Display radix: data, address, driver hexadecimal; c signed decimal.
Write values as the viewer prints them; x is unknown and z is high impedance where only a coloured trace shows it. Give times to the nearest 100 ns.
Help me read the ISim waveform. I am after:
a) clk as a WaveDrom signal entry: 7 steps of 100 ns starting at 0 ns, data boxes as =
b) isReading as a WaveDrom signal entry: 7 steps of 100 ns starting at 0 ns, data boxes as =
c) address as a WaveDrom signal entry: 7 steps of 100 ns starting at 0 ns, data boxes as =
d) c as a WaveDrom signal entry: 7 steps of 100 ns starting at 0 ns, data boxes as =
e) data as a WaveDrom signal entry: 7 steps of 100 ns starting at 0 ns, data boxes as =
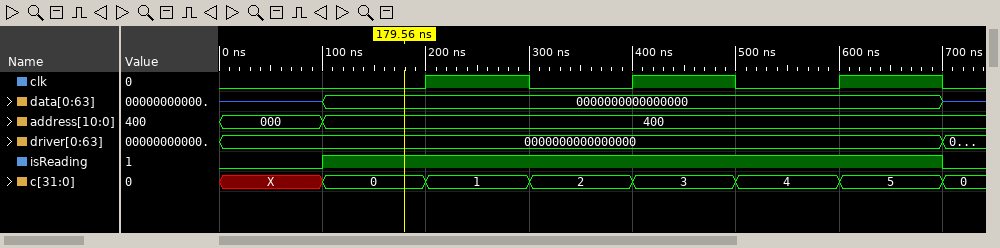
{name: 'clk', wave: '0.10101'}
{name: 'isReading', wave: '01.....'}
{name: 'address', wave: '==.....', data: '000 400'}
{name: 'c', wave: 'x======', data: '0 1 2 3 4 5'}
{name: 'data', wave: 'z=.....', data: '0000000000000000'}
